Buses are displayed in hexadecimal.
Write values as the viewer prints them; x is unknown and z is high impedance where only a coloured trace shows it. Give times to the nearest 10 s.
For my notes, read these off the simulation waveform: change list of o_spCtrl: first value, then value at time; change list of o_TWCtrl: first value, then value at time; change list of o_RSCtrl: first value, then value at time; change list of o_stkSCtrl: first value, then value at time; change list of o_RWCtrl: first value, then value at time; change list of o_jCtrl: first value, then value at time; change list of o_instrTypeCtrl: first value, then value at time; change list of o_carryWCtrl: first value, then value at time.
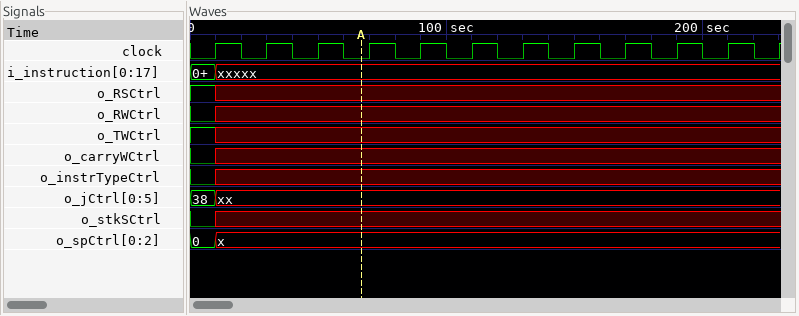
0, x at 10 s
1, x at 10 s
1, x at 10 s
0, x at 10 s
0, x at 10 s
38, xx at 10 s
0, x at 10 s
0, x at 10 s
